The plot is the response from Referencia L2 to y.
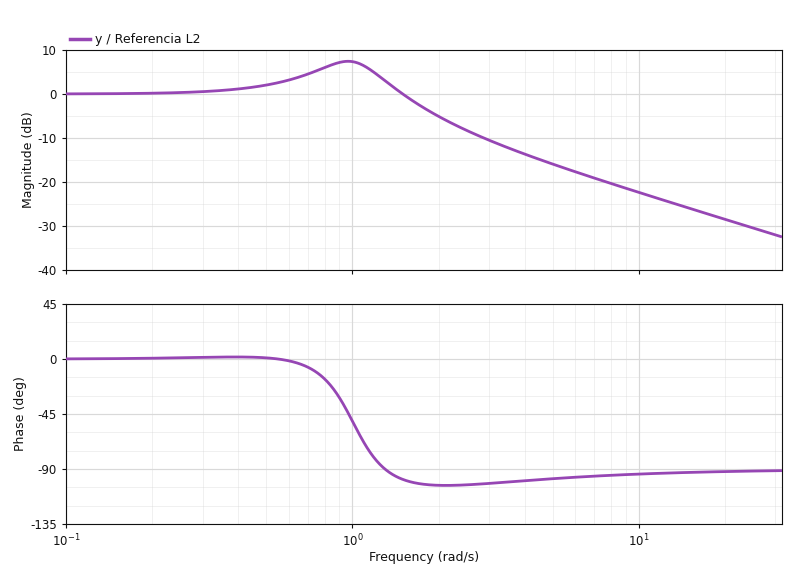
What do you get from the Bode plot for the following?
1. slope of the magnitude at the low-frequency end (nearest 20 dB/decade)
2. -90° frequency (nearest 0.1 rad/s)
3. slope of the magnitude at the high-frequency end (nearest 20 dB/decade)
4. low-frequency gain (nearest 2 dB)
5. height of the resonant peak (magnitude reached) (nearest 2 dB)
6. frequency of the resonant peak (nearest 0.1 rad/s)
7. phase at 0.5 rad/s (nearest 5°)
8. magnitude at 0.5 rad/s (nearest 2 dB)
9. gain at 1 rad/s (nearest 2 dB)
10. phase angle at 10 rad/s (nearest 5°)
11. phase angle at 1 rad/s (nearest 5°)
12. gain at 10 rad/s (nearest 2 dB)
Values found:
0 dB/decade
1.3 rad/s
-20 dB/decade
0 dB
8 dB
1.0 rad/s
0°
2 dB
8 dB
-95°
-50°
-22 dB
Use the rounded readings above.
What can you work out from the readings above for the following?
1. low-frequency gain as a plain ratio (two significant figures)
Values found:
1.0
